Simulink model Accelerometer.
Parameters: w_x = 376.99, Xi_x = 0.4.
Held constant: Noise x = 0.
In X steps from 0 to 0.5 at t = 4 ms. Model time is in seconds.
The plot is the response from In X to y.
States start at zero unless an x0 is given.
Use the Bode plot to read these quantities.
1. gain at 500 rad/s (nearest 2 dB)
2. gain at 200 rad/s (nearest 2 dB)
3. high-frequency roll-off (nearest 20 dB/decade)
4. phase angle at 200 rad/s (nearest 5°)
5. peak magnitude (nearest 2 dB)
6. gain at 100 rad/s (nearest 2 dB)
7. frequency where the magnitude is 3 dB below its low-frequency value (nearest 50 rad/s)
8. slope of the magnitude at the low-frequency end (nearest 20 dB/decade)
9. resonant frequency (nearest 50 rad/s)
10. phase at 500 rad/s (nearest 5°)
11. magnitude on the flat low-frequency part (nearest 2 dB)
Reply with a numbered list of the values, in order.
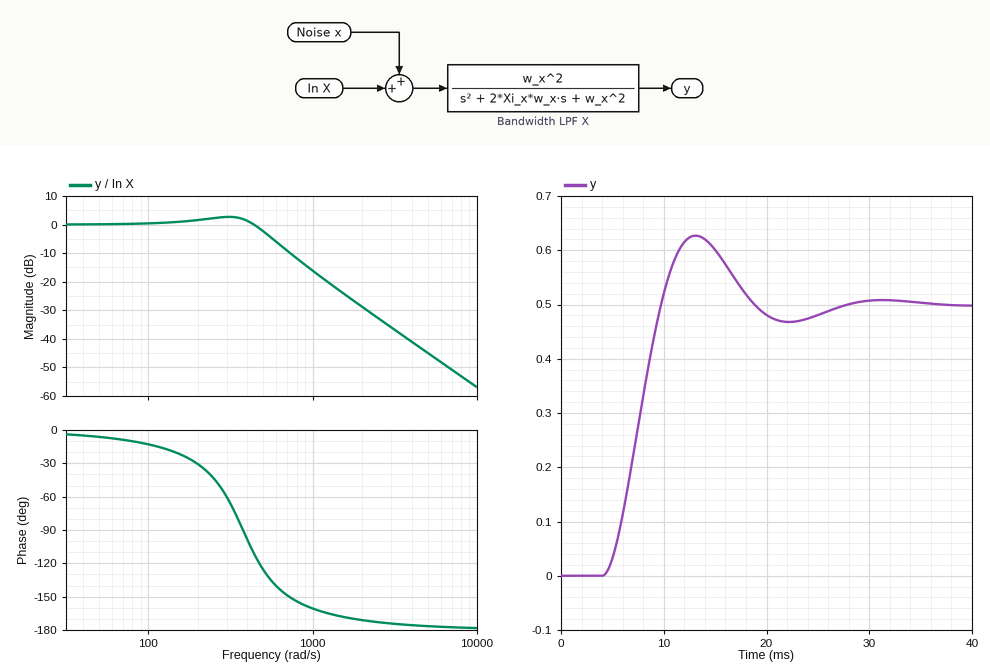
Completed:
1. -2 dB
2. 2 dB
3. -40 dB/decade
4. -30°
5. 2 dB
6. 0 dB
7. 500 rad/s
8. 0 dB/decade
9. 300 rad/s
10. -125°
11. 0 dB
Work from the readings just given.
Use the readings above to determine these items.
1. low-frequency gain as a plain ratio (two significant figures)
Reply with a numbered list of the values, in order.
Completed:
1. 1.0
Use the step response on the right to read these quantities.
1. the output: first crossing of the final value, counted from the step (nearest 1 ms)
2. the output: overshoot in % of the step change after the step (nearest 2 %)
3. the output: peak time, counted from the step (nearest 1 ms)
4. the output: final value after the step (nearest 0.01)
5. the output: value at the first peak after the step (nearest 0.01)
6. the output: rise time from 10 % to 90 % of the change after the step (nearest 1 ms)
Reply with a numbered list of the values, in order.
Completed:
1. 6 ms
2. 26 %
3. 9 ms
4. 0.50
5. 0.63
6. 4 ms
